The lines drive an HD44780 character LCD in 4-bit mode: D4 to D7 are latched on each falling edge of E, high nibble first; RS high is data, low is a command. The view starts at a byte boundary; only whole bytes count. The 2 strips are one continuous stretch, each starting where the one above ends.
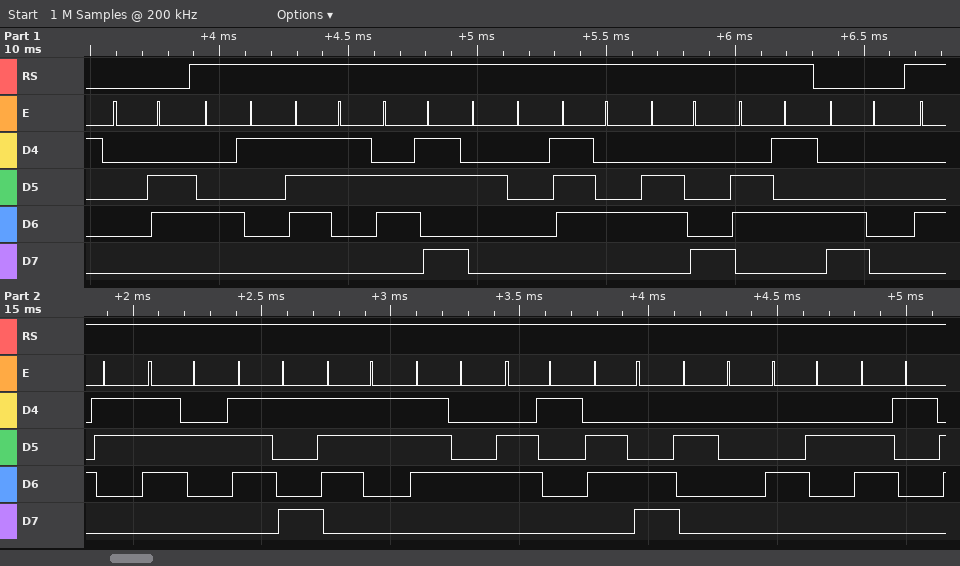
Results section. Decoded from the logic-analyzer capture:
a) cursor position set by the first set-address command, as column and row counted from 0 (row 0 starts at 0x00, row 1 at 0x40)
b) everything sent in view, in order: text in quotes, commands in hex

column 0, row 1
0x06 "Ask the" 0xC0 "Crystal Ba"
